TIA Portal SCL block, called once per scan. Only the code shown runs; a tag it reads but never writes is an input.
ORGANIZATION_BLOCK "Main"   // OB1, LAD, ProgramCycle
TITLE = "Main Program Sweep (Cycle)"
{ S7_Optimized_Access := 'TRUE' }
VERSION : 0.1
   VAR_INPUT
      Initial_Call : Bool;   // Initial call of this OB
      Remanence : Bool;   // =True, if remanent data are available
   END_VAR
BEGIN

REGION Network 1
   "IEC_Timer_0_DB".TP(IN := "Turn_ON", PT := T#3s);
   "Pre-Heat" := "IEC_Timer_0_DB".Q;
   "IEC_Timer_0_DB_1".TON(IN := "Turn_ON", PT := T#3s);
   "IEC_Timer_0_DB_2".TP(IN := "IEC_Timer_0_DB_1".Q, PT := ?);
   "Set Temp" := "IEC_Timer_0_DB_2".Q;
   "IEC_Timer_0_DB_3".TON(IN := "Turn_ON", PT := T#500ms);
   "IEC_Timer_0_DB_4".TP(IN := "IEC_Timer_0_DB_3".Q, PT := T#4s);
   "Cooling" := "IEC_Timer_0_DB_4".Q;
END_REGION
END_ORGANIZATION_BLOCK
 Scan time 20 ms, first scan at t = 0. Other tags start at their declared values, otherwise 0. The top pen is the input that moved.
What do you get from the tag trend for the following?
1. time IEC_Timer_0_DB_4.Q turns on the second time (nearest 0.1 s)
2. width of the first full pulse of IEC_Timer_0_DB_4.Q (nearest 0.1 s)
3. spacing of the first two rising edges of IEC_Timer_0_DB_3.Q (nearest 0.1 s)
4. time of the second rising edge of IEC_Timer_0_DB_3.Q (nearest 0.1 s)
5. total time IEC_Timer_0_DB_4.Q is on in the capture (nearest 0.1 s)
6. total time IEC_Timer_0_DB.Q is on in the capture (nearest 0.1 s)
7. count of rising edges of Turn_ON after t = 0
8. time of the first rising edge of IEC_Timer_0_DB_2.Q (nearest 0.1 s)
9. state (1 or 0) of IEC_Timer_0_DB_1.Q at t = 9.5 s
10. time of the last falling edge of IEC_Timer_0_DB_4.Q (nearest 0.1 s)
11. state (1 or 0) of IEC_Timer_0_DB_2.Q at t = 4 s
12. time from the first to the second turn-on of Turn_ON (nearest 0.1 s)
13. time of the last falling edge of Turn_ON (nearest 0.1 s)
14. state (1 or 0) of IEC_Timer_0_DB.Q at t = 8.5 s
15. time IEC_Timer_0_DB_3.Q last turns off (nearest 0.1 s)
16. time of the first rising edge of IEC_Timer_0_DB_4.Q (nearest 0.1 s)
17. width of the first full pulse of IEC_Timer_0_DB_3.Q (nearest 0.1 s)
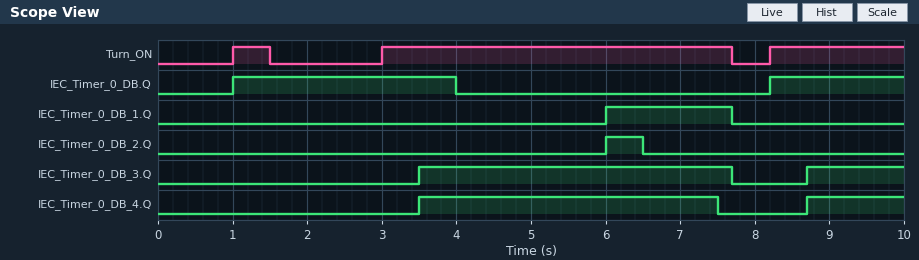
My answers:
8.7 s
4.0 s
5.2 s
8.7 s
5.3 s
4.8 s
3
6.0 s
0
7.5 s
0
2.0 s
7.7 s
1
7.7 s
3.5 s
4.2 s
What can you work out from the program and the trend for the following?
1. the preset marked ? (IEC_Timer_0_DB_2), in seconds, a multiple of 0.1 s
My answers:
0.5 s
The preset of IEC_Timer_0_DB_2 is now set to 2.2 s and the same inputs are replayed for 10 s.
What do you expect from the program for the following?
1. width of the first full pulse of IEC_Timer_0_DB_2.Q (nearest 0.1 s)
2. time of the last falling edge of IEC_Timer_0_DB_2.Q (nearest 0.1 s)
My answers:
2.2 s
8.2 s
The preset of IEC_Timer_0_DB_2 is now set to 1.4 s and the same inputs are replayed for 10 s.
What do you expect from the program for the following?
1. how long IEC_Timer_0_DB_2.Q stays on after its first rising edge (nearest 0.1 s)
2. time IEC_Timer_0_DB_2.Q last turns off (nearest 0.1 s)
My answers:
1.4 s
7.4 s
